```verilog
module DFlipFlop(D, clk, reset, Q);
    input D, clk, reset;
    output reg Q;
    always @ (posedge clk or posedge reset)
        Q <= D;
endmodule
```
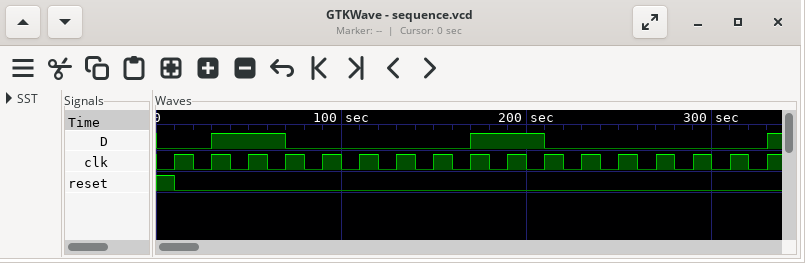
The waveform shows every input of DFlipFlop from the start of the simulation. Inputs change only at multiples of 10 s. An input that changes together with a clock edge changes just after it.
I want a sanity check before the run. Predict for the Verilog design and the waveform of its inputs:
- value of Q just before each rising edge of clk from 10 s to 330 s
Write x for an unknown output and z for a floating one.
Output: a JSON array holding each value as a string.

["0 0 0 1 1 0 0 0 0 0 1 1 0 0 0 0 0"]
